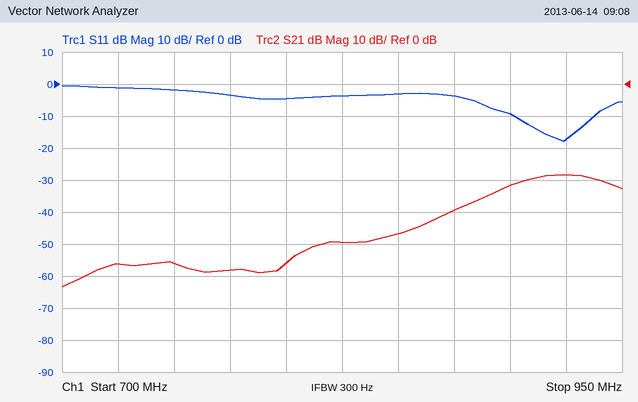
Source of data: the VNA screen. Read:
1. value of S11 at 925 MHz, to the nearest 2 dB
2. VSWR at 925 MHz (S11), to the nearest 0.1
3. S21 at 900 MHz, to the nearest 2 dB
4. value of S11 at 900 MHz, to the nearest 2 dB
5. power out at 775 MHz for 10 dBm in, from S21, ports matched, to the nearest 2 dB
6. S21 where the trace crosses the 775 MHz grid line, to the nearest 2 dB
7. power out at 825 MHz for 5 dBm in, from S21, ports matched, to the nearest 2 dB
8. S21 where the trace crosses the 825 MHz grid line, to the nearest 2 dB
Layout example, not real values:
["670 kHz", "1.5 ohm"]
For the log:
["-18 dB", "1.3", "-32 dB", "-10 dB", "-48 dBm", "-58 dB", "-44 dBm", "-50 dB"]
